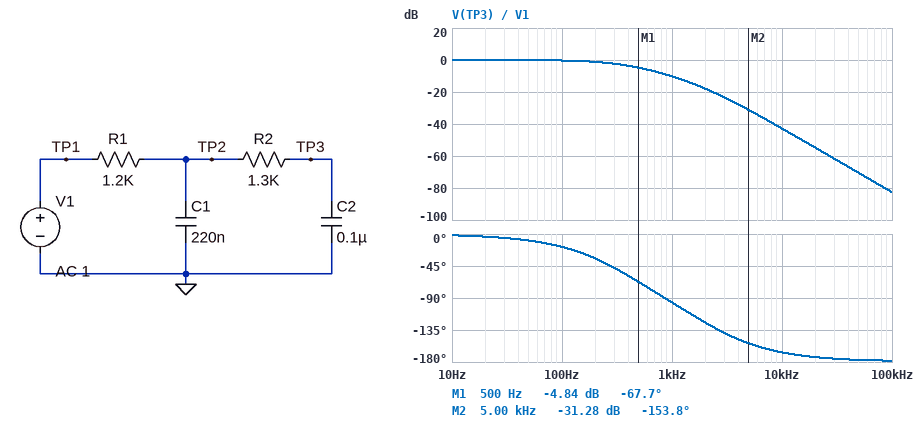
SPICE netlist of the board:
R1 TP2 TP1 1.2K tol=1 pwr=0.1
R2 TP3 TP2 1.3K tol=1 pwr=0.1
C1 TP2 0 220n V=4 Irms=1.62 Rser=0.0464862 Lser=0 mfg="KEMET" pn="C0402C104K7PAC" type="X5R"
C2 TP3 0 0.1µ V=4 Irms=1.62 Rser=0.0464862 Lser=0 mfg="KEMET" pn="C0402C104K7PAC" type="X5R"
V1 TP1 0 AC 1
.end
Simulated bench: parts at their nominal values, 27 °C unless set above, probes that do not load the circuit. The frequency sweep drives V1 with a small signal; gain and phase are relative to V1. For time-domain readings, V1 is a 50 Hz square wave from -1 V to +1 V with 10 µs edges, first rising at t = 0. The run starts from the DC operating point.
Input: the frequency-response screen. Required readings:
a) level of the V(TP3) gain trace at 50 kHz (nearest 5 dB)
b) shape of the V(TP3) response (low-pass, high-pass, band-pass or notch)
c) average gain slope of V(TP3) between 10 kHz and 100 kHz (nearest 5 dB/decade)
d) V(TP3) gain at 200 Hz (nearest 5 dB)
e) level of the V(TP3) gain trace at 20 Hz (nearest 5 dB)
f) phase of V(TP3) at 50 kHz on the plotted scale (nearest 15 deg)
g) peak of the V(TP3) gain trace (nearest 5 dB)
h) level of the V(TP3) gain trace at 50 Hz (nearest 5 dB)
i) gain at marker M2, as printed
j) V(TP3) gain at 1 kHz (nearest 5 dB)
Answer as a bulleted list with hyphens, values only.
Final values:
- -70 dB
- low-pass
- -40 dB/decade
- 0 dB
- 0 dB
- -180 deg
- 0 dB
- 0 dB
- -31.28 dB
- -10 dB
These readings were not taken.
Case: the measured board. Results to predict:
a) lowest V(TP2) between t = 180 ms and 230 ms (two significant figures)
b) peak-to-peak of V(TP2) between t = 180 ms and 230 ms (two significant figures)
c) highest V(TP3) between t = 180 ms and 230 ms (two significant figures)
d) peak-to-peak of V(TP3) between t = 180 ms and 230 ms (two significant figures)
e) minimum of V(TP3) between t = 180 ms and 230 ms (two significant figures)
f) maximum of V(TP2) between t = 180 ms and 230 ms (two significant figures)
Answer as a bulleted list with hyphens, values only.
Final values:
- -1.0 V
- 2.0 V
- 1.0 V
- 2.0 V
- -1.0 V
- 1.0 V
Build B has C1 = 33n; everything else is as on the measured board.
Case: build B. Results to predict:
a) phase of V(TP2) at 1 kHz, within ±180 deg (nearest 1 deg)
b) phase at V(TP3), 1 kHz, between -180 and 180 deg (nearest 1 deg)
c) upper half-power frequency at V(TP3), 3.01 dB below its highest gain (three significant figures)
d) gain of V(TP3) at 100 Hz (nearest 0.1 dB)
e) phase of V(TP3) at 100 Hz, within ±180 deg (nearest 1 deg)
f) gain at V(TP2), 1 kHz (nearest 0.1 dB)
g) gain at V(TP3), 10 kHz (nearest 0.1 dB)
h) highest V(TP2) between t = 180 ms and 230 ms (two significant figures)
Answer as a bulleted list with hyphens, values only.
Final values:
- -27 deg
- -66 deg
- 585 Hz
- -0.1 dB
- -10 deg
- -3.7 dB
- -28.5 dB
- 1.0 V
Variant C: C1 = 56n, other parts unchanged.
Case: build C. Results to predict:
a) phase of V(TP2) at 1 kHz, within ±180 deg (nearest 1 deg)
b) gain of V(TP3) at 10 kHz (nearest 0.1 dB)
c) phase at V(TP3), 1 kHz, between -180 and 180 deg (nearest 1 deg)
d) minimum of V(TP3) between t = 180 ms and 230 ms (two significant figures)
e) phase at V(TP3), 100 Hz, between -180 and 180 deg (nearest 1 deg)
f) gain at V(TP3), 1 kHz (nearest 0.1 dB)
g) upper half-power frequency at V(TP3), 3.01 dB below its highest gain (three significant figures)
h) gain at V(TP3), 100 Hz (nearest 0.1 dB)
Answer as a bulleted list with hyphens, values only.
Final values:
- -33 deg
- -31.8 dB
- -72 deg
- -1.0 V
- -11 deg
- -6.4 dB
- 549 Hz
- -0.1 dB
